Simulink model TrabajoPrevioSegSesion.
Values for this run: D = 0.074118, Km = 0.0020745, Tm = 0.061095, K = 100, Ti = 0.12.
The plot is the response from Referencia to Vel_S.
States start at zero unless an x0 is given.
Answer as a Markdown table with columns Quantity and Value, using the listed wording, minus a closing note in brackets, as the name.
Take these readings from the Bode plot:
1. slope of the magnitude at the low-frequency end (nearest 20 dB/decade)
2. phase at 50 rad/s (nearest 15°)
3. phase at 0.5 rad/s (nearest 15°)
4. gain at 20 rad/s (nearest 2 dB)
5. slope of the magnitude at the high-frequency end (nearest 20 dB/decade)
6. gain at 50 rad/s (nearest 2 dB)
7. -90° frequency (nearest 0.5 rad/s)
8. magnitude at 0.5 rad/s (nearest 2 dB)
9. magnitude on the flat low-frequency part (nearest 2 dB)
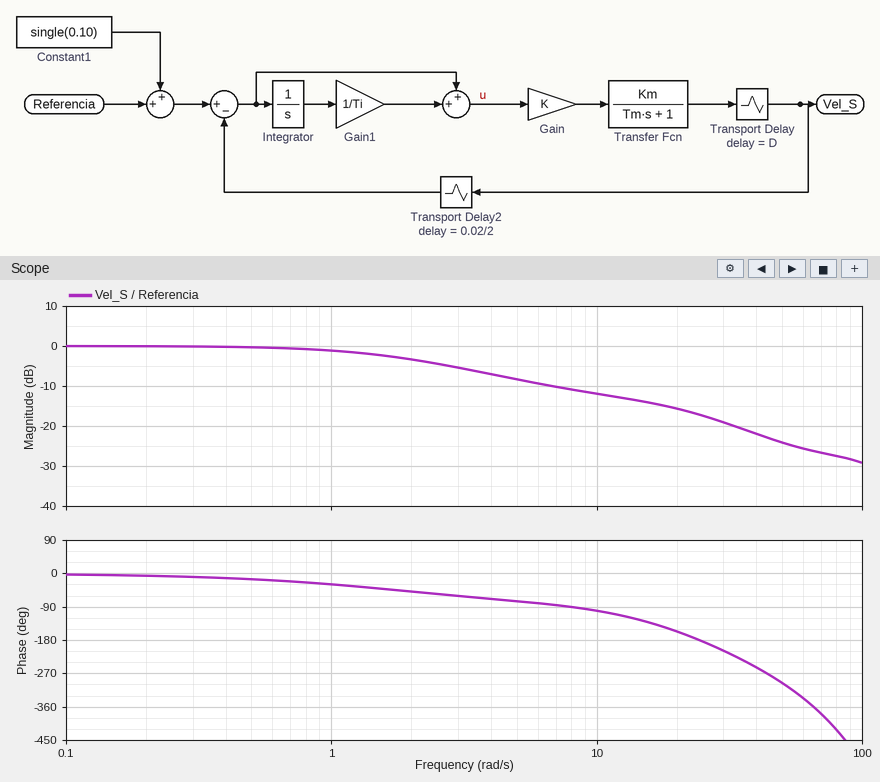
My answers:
| Quantity | Value |
|---|---|
| slope of the magnitude at the low-frequency end | 0 dB/decade |
| phase at 50 rad/s | -300° |
| phase at 0.5 rad/s | -15° |
| gain at 20 rad/s | -16 dB |
| slope of the magnitude at the high-frequency end | -20 dB/decade |
| gain at 50 rad/s | -24 dB |
| -90° frequency | 8.0 rad/s |
| magnitude at 0.5 rad/s | 0 dB |
| magnitude on the flat low-frequency part | 0 dB |
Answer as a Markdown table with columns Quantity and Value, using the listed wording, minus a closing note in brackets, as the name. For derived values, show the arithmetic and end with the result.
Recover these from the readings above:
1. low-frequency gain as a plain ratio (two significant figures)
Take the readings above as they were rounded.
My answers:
| Quantity | Value |
|---|---|
| low-frequency gain as a plain ratio | 10^(0 / 20) = 1.0 |
